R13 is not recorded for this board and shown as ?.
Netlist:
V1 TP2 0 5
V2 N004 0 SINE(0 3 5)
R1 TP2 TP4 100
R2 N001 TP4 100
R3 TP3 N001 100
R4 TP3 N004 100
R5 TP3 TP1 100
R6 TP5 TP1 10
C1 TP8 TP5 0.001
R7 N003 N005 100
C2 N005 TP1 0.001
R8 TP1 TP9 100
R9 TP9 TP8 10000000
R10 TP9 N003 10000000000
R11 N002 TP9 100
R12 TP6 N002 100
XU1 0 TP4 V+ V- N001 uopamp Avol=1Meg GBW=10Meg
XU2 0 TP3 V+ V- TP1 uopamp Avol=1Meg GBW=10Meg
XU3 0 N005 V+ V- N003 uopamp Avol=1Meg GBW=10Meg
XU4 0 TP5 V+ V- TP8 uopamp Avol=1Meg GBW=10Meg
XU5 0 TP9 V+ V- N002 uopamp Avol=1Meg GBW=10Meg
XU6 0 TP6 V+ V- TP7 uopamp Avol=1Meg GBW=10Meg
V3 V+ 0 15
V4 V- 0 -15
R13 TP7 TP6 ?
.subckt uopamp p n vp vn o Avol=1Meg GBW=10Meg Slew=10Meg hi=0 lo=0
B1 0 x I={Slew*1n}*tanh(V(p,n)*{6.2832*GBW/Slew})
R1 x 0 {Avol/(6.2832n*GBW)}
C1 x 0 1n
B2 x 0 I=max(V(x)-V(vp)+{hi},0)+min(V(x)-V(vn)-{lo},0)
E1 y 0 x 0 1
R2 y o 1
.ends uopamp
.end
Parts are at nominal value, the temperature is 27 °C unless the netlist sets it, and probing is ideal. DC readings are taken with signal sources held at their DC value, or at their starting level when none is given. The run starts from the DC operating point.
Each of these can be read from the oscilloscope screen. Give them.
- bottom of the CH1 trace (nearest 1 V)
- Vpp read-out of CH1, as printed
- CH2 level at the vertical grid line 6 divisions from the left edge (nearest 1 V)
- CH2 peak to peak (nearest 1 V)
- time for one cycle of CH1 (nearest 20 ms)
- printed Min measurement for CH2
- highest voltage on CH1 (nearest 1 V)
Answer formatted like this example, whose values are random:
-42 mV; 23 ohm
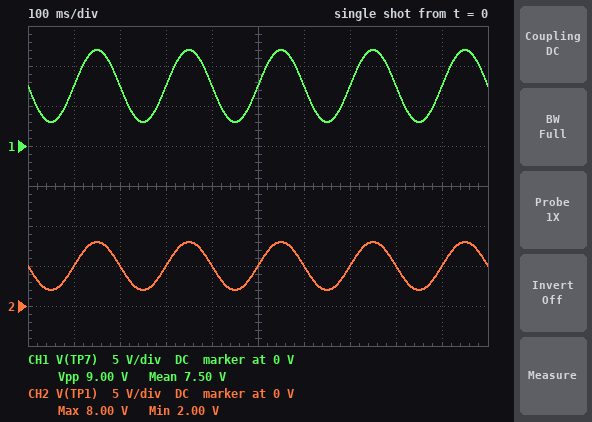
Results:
3 V; 9.00 V; 5 V; 6 V; 200 ms; 2.00 V; 12 V
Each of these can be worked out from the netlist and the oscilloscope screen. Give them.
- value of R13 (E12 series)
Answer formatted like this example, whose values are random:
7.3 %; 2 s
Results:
150 Ω
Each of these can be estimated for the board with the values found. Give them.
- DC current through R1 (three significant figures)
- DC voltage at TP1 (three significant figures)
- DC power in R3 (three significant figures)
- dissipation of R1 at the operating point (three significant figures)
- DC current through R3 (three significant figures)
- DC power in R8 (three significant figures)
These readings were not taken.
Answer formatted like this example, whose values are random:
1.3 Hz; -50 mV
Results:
50.0 mA; 5.00 V; 250 mW; 250 mW; 50.0 mA; 250 mW
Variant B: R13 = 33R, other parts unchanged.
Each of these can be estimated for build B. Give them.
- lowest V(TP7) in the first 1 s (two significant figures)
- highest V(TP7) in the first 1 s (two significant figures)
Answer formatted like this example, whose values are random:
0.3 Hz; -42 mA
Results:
660 mV; 2.6 V
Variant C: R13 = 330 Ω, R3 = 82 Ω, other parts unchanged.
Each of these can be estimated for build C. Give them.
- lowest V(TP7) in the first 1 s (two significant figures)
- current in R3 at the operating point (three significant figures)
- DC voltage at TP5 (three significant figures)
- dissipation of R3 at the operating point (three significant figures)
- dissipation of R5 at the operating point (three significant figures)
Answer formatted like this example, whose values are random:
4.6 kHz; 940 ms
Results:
10 V; 61.0 mA; 6.10 V; 305 mW; 372 mW
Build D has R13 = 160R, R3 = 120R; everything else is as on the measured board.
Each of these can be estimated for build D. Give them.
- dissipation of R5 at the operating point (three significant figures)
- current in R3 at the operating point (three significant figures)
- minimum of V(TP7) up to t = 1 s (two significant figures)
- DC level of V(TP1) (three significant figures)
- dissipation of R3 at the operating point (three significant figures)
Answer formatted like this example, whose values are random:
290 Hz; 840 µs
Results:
174 mW; 41.7 mA; 1.9 V; 4.17 V; 208 mW
